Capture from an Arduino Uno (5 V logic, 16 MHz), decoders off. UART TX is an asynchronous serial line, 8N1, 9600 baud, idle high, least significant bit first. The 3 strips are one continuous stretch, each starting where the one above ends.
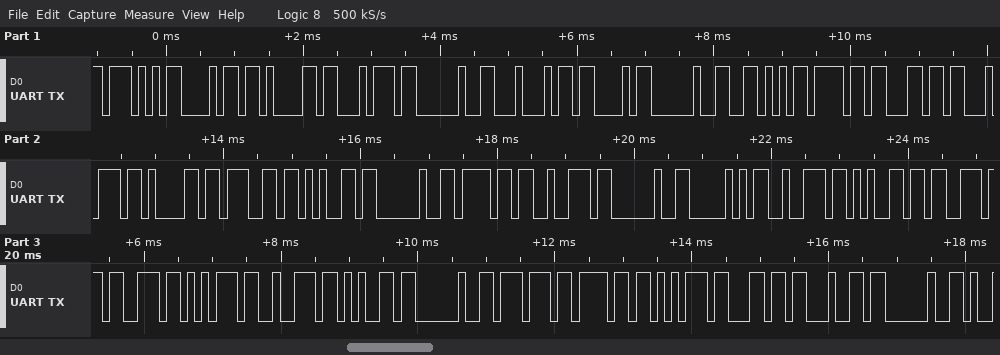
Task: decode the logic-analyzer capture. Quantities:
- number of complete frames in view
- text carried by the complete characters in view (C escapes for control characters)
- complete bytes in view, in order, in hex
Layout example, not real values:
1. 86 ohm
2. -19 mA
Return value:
1. 34
2. "What DC Voltage or Pressure would "
3. 57 68 61 74 20 44 43 20 56 6F 6C 74 61 67 65 20 6F 72 20 50 72 65 73 73 75 72 65 20 77 6F 75 6C 64 20
